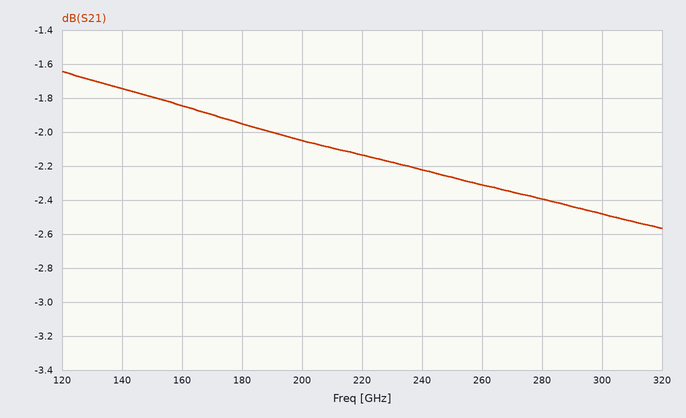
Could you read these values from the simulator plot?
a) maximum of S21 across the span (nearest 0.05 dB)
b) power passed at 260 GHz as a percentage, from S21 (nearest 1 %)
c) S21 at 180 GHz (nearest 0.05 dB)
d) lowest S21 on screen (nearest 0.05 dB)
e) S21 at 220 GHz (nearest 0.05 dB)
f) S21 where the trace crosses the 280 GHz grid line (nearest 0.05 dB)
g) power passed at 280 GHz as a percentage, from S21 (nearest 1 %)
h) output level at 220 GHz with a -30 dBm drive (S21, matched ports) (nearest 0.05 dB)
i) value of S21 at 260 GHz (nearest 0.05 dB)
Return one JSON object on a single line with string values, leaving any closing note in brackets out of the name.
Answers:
{"maximum of S21 across the span": "-1.65 dB", "power passed at 260 GHz as a percentage, from S21": "59 %", "S21 at 180 GHz": "-1.95 dB", "lowest S21 on screen": "-2.55 dB", "S21 at 220 GHz": "-2.15 dB", "S21 where the trace crosses the 280 GHz grid line": "-2.40 dB", "power passed at 280 GHz as a percentage, from S21": "58 %", "output level at 220 GHz with a -30 dBm drive (S21, matched ports)": "-32.15 dBm", "value of S21 at 260 GHz": "-2.30 dB"}
